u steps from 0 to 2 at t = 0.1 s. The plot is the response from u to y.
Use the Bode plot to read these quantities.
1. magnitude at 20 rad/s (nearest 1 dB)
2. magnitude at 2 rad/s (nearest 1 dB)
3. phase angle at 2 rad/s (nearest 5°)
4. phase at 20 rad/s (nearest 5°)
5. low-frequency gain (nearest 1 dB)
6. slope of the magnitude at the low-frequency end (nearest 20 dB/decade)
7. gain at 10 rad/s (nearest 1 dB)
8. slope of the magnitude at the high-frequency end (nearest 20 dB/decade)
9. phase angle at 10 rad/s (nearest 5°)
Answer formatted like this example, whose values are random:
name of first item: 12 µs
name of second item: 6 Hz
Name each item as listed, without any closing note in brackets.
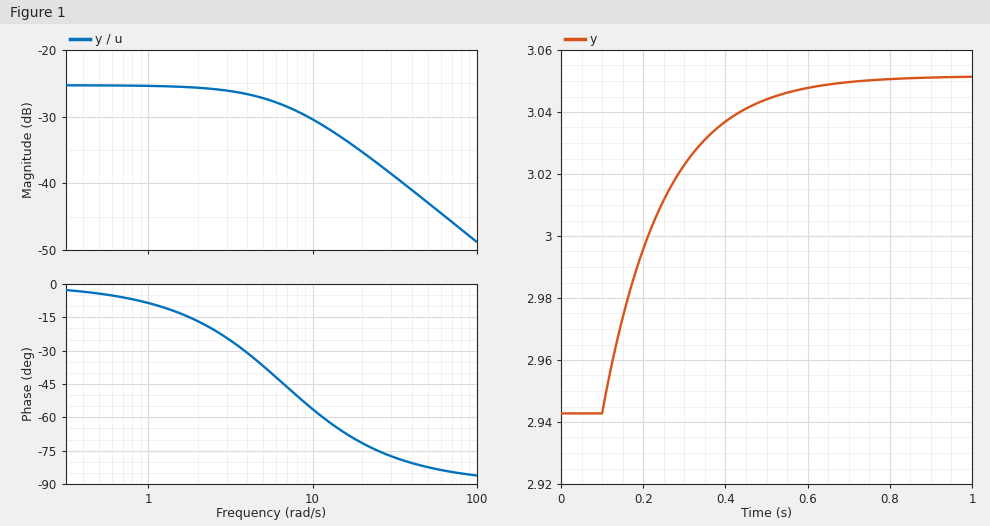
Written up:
magnitude at 20 rad/s: -35 dB
magnitude at 2 rad/s: -26 dB
phase angle at 2 rad/s: -15°
phase at 20 rad/s: -70°
low-frequency gain: -25 dB
slope of the magnitude at the low-frequency end: 0 dB/decade
gain at 10 rad/s: -30 dB
slope of the magnitude at the high-frequency end: -20 dB/decade
phase angle at 10 rad/s: -55°
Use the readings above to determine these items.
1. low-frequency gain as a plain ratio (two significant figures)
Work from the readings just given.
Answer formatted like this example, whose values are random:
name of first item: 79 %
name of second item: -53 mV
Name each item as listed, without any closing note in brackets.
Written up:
low-frequency gain as a plain ratio: 0.056
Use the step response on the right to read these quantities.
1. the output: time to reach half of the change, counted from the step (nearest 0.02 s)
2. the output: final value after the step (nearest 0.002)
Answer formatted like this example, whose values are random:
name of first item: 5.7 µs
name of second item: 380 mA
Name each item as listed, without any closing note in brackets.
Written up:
the output: time to reach half of the change, counted from the step: 0.10 s
the output: final value after the step: 3.052
